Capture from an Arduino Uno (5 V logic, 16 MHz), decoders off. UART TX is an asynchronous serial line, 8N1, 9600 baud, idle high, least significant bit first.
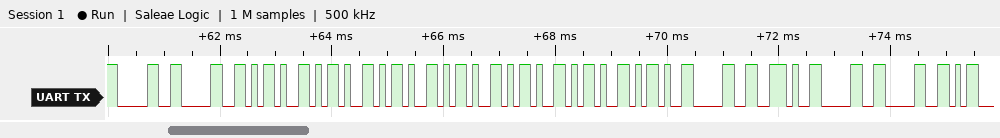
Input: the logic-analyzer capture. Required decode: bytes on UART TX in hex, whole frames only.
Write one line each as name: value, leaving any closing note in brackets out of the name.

bytes on UART TX in hex, whole frames only: 0x30 0x30 0x2D 0x2D 0x2D 0x2D 0x2D 0x2D 0x2D 0x30 0x2E 0x30 0x30
